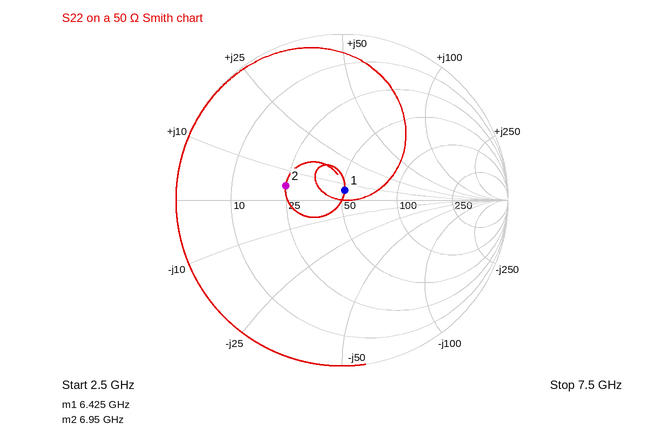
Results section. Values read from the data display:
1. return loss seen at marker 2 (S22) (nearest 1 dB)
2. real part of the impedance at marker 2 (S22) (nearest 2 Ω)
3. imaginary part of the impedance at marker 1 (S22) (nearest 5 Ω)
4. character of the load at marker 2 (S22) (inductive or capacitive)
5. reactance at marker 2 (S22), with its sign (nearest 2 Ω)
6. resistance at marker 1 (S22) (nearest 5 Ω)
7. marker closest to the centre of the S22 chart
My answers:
9 dB
24 Ω
+5 Ω
inductive
+4 Ω
50 Ω
marker 1
